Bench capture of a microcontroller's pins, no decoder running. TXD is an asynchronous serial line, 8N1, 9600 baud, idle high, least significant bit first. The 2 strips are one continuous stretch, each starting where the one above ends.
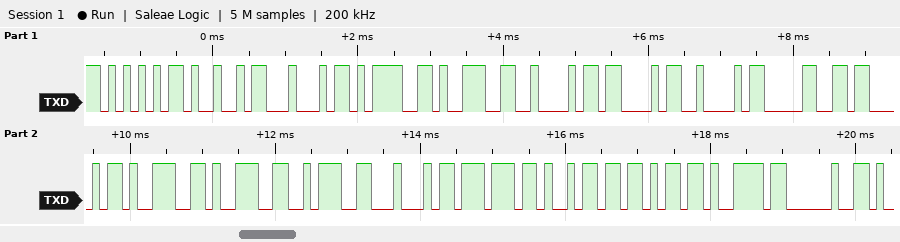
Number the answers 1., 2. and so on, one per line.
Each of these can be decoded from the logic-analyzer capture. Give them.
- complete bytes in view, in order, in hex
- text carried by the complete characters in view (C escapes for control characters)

1. 0x55 0x49 0x44 0x3D 0x39 0x42 0x43 0x42 0x30 0x43 0x39 0x39 0x3A 0x44 0x77 0x69 0x6B 0x79 0x20
2. "UID=9BCB0C99:Dwiky "
